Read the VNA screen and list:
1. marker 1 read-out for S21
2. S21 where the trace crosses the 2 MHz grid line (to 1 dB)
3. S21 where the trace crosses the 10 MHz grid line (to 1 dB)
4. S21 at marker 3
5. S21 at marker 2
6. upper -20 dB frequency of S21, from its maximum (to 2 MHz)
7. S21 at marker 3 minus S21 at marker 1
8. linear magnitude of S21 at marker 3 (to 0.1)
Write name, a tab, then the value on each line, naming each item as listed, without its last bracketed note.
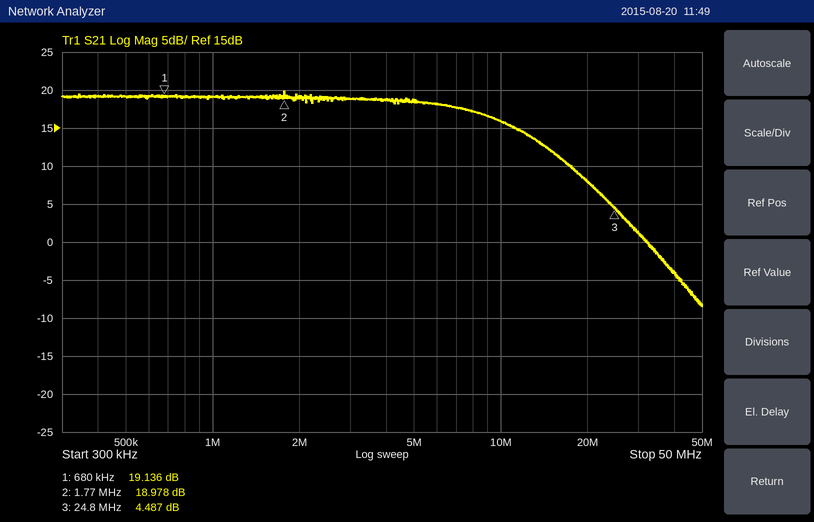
marker 1 read-out for S21	19.136 dB
S21 where the trace crosses the 2 MHz grid line	19 dB
S21 where the trace crosses the 10 MHz grid line	16 dB
S21 at marker 3	4.487 dB
S21 at marker 2	18.978 dB
upper -20 dB frequency of S21, from its maximum	32 MHz
S21 at marker 3 minus S21 at marker 1	-14.649 dB
linear magnitude of S21 at marker 3	1.7
